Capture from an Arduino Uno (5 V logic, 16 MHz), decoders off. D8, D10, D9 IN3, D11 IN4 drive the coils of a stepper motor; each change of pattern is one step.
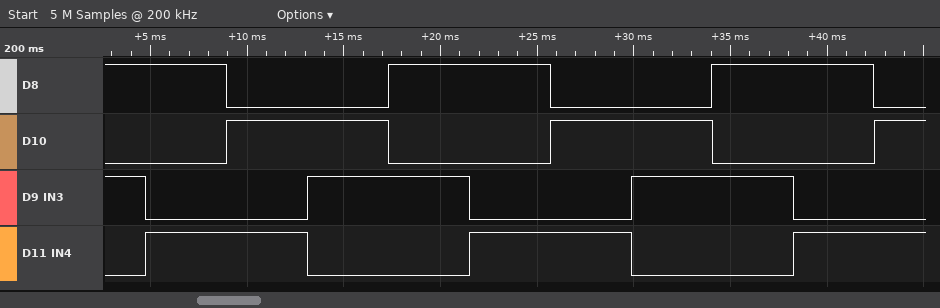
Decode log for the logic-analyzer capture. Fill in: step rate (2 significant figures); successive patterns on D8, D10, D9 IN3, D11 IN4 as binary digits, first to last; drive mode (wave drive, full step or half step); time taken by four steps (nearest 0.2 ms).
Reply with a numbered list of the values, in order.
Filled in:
1. 240 steps/s
2. 1010 1001 0101 0110 1010 1001 0101 0110 1010 1001 0101
3. full step
4. 16.8 ms
